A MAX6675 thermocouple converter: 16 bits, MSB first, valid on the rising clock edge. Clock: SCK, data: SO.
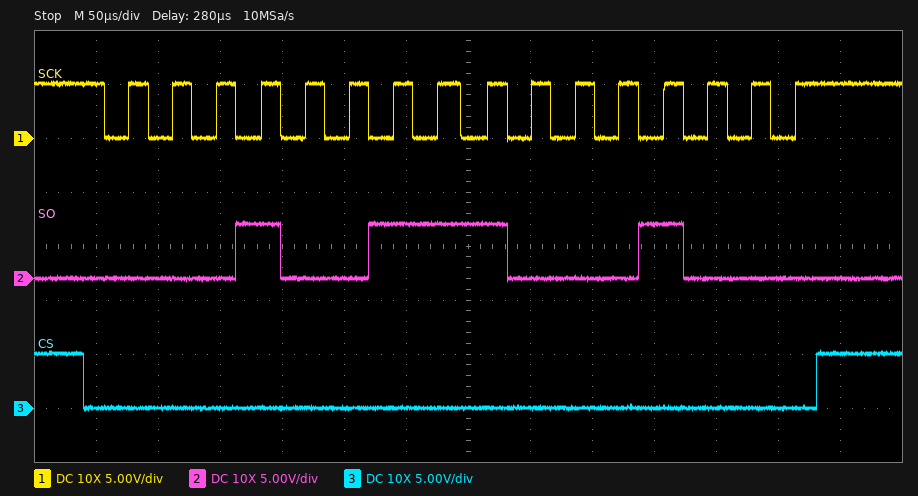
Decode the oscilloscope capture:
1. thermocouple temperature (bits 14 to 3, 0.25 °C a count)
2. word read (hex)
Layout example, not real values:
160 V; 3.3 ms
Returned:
156.25 °C; 0x1388
